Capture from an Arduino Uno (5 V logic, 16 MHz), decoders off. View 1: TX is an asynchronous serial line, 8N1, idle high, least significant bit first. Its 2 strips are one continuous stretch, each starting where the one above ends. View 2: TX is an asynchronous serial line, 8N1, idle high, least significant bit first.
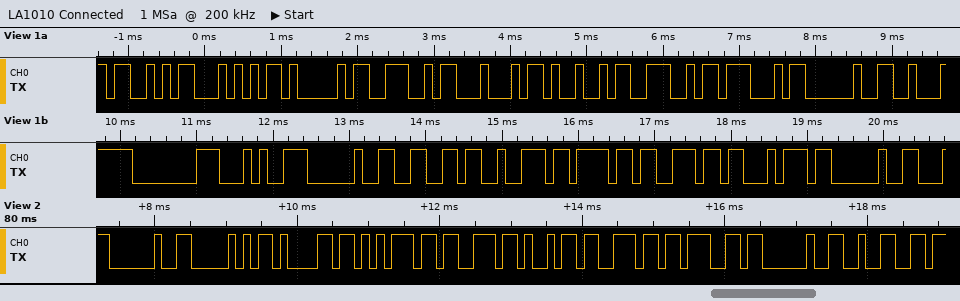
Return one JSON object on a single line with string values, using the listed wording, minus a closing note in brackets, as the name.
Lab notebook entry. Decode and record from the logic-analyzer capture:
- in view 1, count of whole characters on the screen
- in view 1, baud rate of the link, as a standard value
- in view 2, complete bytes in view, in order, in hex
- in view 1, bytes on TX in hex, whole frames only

{"in view 1, count of whole characters on the screen": "19", "in view 1, baud rate of the link, as a standard value": "9600 baud", "in view 2, complete bytes in view, in order, in hex": "20 50 61 75 73 69 6E 67 20 32", "in view 1, bytes on TX in hex, whole frames only": "0x53 0x54 0x41 0x4E 0x44 0x49 0x4E 0x47 0x20 0xE2 0x80 0x94 0x20 0x66 0x72 0x6F 0x6E 0x74 0x20"}
